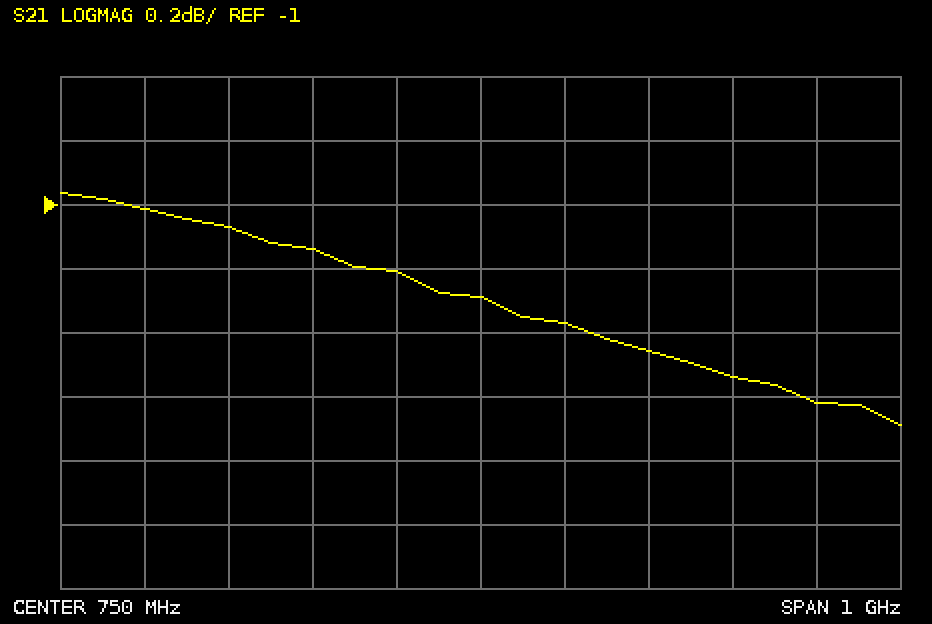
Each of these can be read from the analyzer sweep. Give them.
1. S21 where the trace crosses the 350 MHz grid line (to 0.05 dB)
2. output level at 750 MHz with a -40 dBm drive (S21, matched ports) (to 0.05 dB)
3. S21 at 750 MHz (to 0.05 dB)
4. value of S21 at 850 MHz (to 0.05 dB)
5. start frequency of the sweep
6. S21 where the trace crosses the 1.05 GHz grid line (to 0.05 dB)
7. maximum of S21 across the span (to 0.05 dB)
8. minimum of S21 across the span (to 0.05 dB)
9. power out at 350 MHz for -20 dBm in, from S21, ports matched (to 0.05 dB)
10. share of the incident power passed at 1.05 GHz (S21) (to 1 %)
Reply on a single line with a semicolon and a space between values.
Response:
-1.00 dB; -41.30 dBm; -1.30 dB; -1.35 dB; 250 MHz; -1.55 dB; -0.95 dB; -1.70 dB; -21.00 dBm; 70 %
